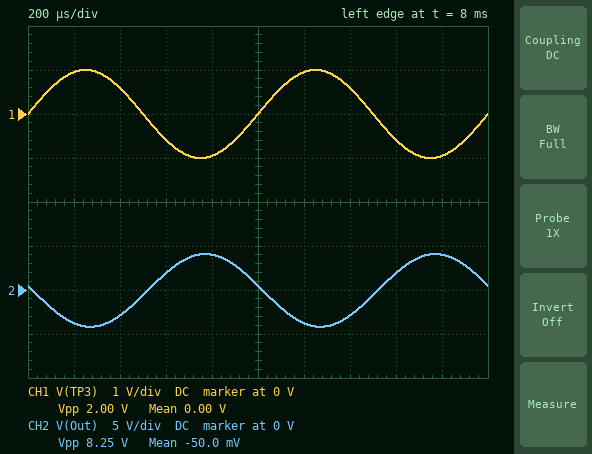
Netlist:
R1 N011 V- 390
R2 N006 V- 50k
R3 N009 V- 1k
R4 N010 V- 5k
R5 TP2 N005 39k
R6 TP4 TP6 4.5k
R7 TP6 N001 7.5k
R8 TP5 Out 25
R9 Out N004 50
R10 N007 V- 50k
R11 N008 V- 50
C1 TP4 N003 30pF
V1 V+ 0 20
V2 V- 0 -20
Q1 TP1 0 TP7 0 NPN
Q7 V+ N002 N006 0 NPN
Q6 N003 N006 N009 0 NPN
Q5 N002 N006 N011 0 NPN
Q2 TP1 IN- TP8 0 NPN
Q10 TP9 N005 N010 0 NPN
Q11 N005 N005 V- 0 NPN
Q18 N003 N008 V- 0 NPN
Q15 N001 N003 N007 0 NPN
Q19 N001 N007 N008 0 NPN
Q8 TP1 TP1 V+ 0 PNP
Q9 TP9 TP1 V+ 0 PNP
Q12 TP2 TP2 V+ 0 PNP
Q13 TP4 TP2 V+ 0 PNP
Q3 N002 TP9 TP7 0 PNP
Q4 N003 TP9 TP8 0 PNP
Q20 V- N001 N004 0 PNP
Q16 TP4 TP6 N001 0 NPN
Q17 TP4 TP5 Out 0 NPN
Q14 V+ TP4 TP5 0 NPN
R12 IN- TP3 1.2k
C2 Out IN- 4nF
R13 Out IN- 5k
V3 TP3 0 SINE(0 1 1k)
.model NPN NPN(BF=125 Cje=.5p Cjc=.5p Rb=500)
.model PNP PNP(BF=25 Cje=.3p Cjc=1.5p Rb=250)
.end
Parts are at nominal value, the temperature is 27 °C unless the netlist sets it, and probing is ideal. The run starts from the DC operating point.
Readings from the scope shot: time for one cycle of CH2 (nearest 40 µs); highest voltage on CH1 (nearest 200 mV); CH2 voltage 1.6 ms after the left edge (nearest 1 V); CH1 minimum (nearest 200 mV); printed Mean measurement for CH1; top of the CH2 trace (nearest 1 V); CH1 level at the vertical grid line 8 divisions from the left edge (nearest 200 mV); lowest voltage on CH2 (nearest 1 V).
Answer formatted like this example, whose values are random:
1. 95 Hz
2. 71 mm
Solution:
1. 1.00 ms
2. 1.0 V
3. 2 V
4. -1.0 V
5. 0.00 V
6. 4 V
7. -600 mV
8. -4 V
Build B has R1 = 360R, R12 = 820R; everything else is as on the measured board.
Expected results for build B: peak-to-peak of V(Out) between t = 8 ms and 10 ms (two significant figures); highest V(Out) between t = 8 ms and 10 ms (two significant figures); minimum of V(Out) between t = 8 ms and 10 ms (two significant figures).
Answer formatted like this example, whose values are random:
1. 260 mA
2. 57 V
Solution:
1. 12 V
2. 6.0 V
3. -6.1 V
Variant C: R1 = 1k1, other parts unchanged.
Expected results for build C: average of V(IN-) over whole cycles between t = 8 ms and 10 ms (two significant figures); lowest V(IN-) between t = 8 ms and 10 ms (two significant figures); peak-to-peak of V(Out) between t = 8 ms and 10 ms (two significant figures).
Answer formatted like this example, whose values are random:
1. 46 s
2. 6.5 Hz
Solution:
1. 1.8 mV
2. -4.3 mV
3. 8.3 V
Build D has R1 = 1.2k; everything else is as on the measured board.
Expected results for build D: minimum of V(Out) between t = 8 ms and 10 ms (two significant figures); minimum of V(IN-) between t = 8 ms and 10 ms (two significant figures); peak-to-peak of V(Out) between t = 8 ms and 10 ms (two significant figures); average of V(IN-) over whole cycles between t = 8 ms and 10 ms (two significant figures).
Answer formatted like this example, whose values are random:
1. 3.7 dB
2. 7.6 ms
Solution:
1. -4.1 V
2. -2.8 mV
3. 8.3 V
4. 3.2 mV
